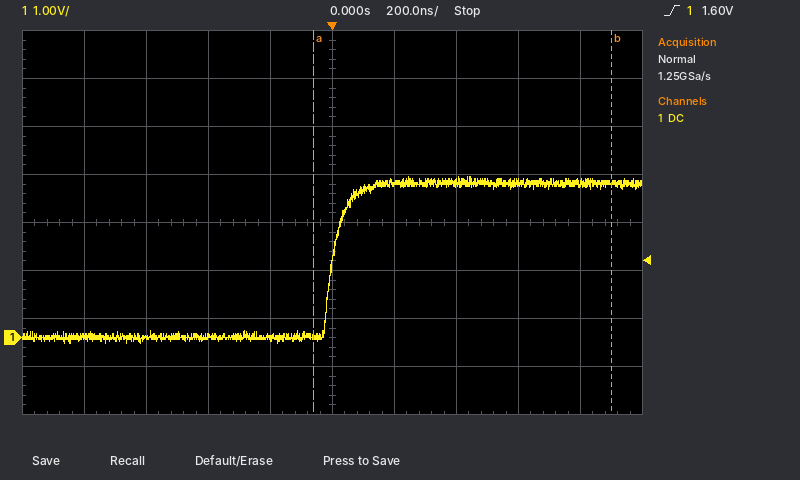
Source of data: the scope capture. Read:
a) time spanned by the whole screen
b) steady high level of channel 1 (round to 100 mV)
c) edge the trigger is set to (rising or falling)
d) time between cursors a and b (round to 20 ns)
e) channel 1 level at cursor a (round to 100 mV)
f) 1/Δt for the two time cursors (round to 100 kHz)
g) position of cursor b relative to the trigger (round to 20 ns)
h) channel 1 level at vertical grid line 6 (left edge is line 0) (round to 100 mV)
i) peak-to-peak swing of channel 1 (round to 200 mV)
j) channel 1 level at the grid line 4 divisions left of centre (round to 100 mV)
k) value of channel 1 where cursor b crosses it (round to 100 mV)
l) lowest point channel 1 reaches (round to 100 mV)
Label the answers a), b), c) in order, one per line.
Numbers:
a) 2 µs
b) 3.2 V
c) rising
d) 960 ns
e) 0.0 V
f) 1.0 MHz
g) +900 ns
h) 3.2 V
i) 3.4 V
j) 0.0 V
k) 3.2 V
l) -100 mV
